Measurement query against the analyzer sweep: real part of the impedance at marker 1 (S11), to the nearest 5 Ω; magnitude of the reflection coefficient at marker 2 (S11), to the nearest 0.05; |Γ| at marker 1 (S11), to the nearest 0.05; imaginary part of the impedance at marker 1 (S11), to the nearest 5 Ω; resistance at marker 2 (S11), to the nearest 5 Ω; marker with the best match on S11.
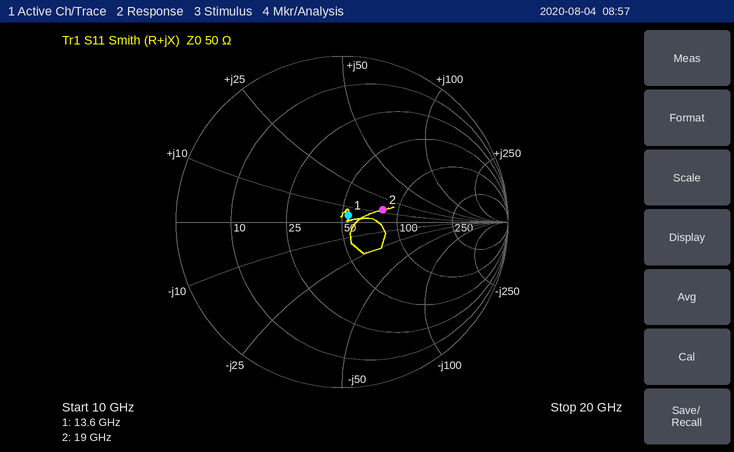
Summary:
55 Ω
0.25
0.05
+5 Ω
80 Ω
marker 1
